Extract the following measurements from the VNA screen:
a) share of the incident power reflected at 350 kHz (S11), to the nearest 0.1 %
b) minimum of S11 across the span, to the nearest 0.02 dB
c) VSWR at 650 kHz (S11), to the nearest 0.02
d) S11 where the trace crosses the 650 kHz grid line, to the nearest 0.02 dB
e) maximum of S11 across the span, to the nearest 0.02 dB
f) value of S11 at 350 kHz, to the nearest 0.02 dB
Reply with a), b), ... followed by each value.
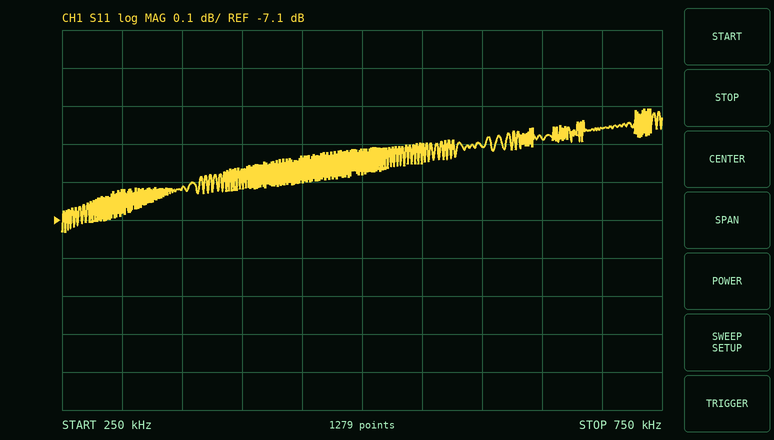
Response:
a) 19.9 %
b) -7.14 dB
c) 2.66
d) -6.88 dB
e) -6.80 dB
f) -7.02 dB
